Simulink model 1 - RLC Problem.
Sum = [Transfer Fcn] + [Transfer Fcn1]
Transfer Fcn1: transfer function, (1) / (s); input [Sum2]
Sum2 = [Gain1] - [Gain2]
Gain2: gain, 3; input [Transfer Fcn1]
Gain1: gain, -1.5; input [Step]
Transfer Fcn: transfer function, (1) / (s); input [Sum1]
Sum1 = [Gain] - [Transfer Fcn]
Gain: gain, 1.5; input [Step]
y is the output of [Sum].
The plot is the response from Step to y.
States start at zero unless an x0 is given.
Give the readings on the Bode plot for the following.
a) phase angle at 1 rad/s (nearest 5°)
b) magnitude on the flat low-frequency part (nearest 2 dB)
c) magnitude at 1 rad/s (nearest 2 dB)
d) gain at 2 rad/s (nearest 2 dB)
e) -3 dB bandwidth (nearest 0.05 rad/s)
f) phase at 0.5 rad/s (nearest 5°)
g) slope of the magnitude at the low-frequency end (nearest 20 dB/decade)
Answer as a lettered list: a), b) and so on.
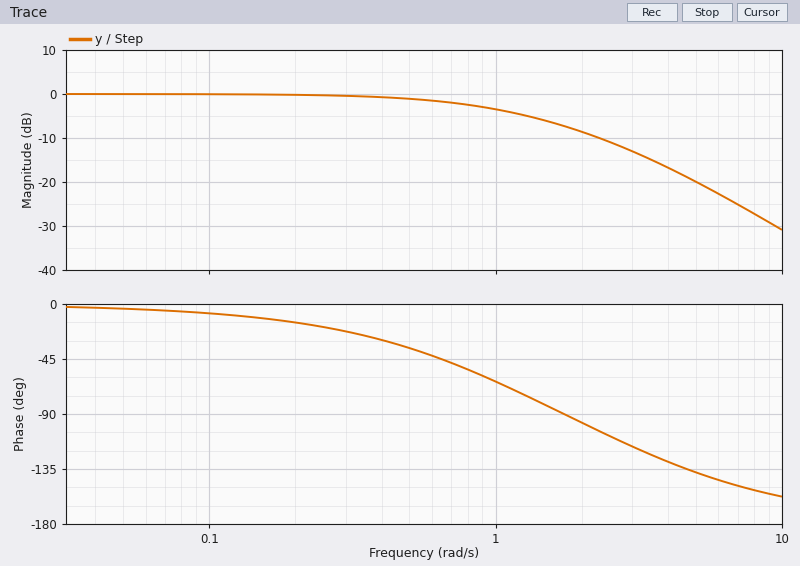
a) -65°
b) 0 dB
c) -4 dB
d) -8 dB
e) 0.90 rad/s
f) -35°
g) 0 dB/decade
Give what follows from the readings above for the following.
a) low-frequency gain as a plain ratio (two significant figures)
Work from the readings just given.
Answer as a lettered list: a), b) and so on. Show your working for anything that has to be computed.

a) 10^(0 / 20) = 1.0
